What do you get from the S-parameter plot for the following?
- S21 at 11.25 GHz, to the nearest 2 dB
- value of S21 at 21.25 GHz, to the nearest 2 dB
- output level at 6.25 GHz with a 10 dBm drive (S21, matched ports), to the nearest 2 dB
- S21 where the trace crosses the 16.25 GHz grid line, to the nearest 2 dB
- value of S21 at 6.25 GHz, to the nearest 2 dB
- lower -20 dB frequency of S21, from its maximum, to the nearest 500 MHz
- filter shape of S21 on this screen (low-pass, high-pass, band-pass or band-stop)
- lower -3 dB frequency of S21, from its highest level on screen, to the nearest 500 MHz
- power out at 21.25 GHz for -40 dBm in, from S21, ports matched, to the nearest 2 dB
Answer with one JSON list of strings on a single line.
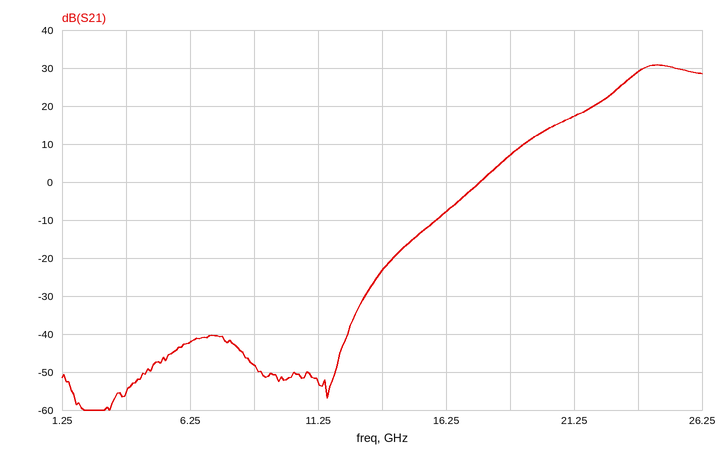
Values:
["-52 dB", "18 dB", "-32 dBm", "-8 dB", "-42 dB", "19.5 GHz", "high-pass", "23.5 GHz", "-22 dBm"]
